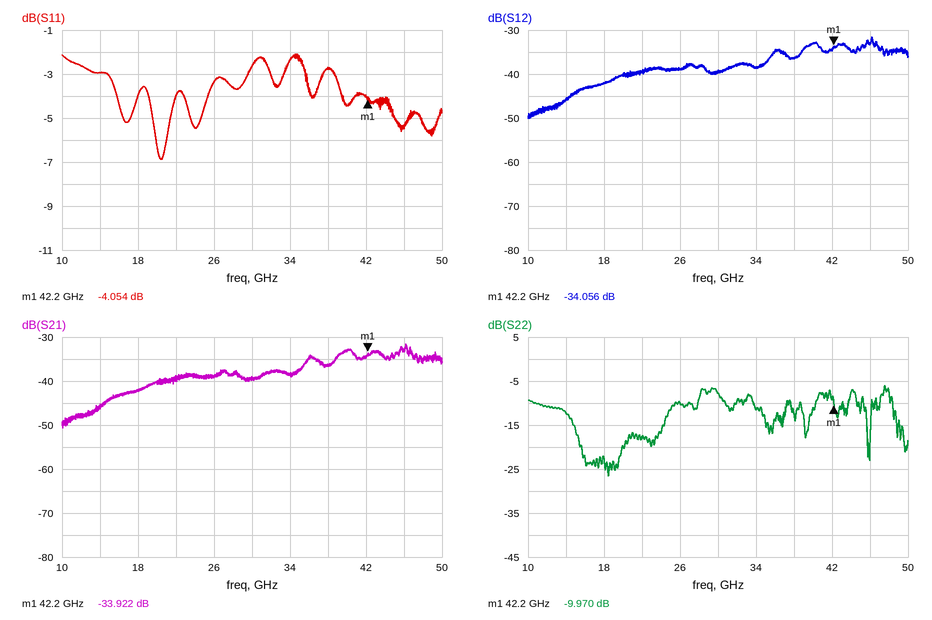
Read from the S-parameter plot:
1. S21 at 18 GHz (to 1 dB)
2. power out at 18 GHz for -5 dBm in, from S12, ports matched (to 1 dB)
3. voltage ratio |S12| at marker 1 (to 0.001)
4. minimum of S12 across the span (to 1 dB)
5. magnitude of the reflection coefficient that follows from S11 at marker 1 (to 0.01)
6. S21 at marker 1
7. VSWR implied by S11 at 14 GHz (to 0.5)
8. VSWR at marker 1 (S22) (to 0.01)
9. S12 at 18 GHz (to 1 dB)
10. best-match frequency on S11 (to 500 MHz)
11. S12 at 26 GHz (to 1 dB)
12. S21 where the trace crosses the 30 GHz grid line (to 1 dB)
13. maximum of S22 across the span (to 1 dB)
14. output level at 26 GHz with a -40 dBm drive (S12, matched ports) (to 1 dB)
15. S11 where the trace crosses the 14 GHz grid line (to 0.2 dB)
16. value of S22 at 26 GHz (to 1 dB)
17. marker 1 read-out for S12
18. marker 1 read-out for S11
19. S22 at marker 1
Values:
-42 dB
-47 dBm
0.020
-50 dB
0.63
-33.922 dB
6.0
1.93
-42 dB
20.5 GHz
-39 dB
-39 dB
-6 dB
-79 dBm
-3.0 dB
-10 dB
-34.056 dB
-4.054 dB
-9.970 dB
